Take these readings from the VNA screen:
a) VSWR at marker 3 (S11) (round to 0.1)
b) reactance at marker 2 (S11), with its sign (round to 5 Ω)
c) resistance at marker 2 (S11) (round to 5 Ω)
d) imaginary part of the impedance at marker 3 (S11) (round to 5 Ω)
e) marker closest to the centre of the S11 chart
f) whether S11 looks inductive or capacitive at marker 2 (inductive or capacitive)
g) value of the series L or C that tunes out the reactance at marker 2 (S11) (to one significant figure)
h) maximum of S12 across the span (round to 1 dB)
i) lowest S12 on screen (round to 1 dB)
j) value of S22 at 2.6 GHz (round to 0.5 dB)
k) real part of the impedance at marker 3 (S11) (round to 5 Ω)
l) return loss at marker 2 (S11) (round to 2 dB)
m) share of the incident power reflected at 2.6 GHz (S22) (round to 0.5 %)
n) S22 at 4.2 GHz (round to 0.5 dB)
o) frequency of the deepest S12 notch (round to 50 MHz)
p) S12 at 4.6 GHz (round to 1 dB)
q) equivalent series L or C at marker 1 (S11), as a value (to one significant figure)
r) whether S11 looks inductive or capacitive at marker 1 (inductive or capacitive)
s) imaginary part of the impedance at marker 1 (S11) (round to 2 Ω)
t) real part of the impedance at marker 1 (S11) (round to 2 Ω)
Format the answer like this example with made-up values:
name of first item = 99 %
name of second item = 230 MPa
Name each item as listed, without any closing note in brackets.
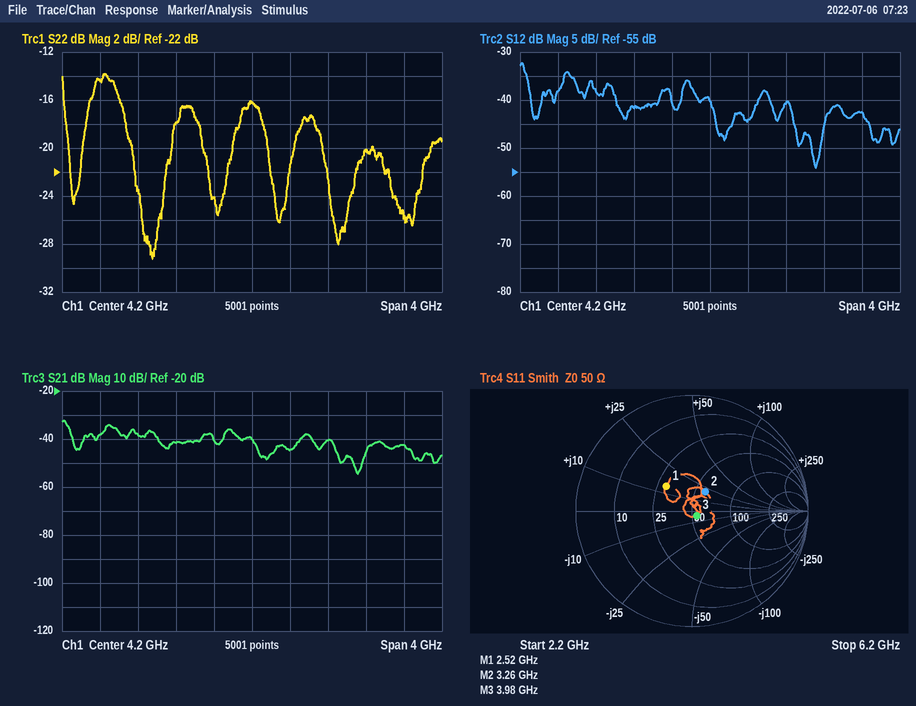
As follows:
VSWR at marker 3 (S11) = 1.1
reactance at marker 2 (S11), with its sign = +20 Ω
resistance at marker 2 (S11) = 60 Ω
imaginary part of the impedance at marker 3 (S11) = -5 Ω
marker closest to the centre of the S11 chart = marker 3
whether S11 looks inductive or capacitive at marker 2 = inductive
value of the series L or C that tunes out the reactance at marker 2 (S11) = 2 pF
maximum of S12 across the span = -32 dB
lowest S12 on screen = -54 dB
value of S22 at 2.6 GHz = -14.5 dB
real part of the impedance at marker 3 (S11) = 55 Ω
return loss at marker 2 (S11) = 14 dB
share of the incident power reflected at 2.6 GHz (S22) = 3.5 %
S22 at 4.2 GHz = -16.0 dB
frequency of the deepest S12 notch = 5.30 GHz
S12 at 4.6 GHz = -44 dB
equivalent series L or C at marker 1 (S11), as a value = 900 pH
whether S11 looks inductive or capacitive at marker 1 = inductive
imaginary part of the impedance at marker 1 (S11) = +14 Ω
real part of the impedance at marker 1 (S11) = 30 Ω
